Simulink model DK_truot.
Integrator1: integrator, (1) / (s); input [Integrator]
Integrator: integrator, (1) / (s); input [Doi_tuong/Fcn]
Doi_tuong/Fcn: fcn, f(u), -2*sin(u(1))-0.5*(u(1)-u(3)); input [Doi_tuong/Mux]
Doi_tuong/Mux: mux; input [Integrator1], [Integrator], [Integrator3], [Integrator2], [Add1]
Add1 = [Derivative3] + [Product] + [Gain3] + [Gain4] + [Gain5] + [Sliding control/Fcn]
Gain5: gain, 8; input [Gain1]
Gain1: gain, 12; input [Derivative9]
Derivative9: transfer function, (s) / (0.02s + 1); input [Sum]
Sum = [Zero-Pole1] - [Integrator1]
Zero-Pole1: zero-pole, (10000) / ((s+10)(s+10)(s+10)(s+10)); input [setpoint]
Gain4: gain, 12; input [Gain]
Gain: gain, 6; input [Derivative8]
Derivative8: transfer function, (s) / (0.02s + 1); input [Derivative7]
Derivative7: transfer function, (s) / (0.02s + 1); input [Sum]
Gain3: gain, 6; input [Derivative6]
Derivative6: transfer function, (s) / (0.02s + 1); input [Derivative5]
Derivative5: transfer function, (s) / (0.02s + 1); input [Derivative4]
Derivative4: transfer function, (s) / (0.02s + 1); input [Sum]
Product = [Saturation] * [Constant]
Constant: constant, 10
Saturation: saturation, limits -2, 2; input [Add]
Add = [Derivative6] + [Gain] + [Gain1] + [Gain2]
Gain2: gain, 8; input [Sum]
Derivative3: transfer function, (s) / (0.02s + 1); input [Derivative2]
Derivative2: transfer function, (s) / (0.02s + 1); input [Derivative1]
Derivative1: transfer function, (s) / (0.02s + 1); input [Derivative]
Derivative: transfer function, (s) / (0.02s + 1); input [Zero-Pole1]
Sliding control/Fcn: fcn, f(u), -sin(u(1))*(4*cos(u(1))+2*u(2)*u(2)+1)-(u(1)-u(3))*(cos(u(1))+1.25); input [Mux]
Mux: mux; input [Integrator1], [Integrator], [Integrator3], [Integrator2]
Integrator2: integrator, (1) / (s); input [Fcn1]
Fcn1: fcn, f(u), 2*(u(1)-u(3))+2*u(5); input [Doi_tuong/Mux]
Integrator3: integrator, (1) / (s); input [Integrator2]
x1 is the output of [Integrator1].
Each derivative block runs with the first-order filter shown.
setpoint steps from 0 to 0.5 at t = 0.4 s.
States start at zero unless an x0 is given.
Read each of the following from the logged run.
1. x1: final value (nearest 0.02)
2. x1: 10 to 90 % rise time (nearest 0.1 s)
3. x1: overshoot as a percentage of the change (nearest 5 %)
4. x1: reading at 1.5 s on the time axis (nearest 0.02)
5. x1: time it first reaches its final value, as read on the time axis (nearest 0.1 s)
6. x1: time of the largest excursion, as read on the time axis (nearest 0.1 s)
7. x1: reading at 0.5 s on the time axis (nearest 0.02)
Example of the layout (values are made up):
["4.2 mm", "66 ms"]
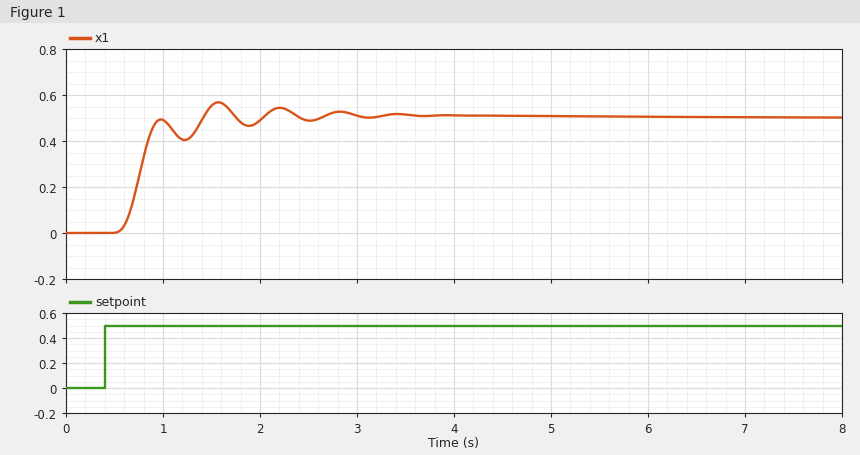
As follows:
["0.50", "0.3 s", "15 %", "0.56", "1.4 s", "1.6 s", "0.00"]
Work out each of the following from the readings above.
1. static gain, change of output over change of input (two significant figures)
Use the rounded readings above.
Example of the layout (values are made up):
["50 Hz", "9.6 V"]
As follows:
["1.0"]
